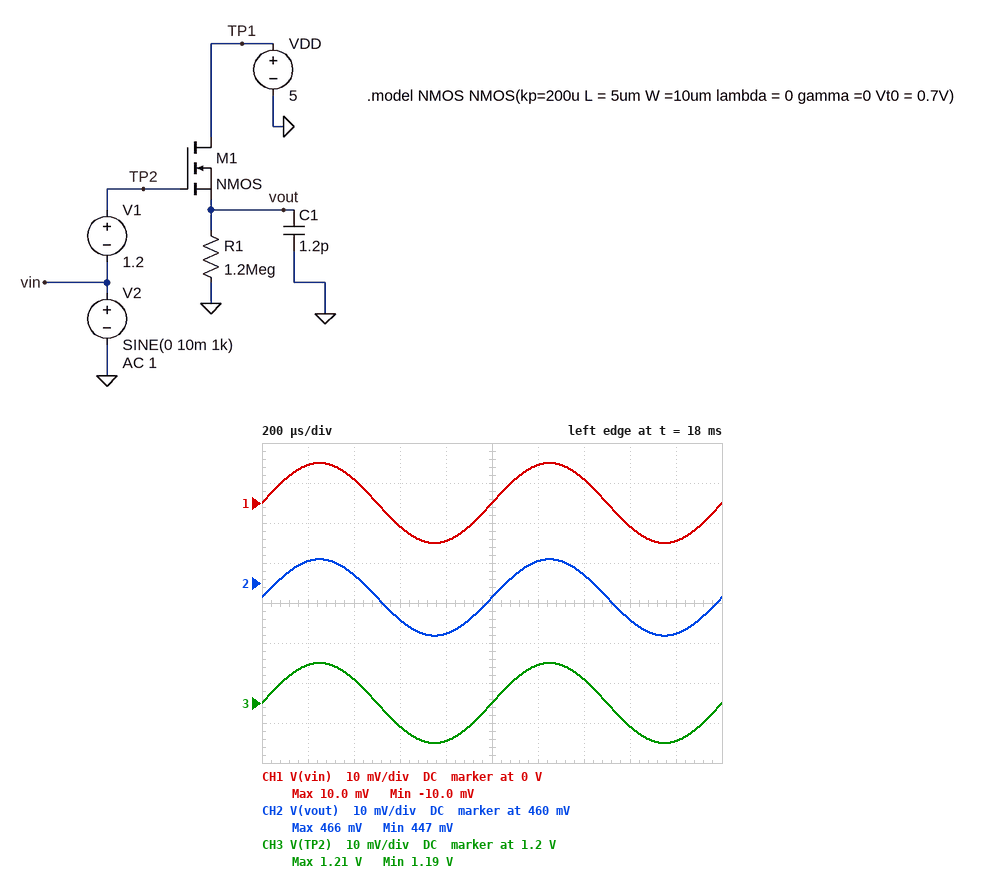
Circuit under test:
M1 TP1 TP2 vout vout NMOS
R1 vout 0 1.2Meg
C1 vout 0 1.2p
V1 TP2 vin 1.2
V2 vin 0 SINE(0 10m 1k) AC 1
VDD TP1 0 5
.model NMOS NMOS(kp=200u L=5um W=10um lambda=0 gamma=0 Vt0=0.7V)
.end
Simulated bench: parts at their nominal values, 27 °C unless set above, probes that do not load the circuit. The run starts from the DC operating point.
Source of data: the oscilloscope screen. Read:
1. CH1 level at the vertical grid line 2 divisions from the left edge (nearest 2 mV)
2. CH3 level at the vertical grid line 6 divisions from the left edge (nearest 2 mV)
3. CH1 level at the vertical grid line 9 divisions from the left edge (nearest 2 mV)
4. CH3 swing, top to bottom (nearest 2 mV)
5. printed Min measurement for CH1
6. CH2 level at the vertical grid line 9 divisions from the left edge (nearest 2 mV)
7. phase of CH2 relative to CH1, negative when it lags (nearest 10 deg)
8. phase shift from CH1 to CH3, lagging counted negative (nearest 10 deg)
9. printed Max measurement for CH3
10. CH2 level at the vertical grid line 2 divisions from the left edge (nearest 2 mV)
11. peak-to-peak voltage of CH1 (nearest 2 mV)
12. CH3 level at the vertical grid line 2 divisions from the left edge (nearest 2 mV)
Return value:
6 mV
1.210 V
-10 mV
20 mV
-10.0 mV
448 mV
0 deg
0 deg
1.21 V
462 mV
20 mV
1.206 V
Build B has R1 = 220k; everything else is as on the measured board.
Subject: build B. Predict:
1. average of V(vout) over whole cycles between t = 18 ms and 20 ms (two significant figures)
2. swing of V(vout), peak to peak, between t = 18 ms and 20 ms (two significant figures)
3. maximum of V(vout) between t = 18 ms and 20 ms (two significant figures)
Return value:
400 mV
18 mV
410 mV
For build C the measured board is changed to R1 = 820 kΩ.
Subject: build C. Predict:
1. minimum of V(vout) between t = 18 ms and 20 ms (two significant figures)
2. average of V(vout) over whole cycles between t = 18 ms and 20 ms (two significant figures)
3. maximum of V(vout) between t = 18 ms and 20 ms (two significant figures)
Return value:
440 mV
450 mV
460 mV
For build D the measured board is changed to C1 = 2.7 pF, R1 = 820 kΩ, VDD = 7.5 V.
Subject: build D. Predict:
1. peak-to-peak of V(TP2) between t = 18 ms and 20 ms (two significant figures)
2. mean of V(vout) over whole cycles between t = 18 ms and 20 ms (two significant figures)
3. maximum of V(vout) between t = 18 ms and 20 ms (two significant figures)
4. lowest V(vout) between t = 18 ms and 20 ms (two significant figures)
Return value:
20 mV
450 mV
460 mV
440 mV
